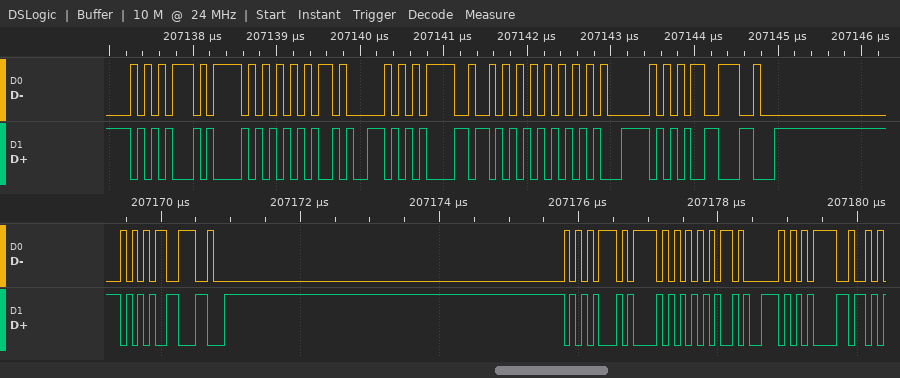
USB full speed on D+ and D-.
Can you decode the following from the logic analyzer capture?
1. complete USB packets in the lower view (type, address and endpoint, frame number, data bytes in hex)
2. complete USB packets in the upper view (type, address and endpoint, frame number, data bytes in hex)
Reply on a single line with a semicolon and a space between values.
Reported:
NAK, OUT ADDR 0 EP 0; OUT ADDR 0 EP 0, DATA1 [ ], NAK
